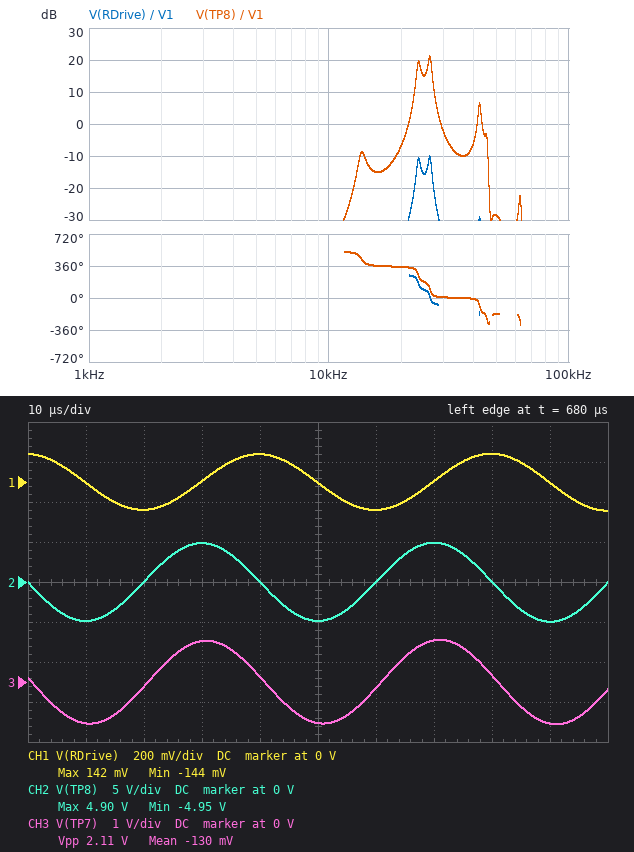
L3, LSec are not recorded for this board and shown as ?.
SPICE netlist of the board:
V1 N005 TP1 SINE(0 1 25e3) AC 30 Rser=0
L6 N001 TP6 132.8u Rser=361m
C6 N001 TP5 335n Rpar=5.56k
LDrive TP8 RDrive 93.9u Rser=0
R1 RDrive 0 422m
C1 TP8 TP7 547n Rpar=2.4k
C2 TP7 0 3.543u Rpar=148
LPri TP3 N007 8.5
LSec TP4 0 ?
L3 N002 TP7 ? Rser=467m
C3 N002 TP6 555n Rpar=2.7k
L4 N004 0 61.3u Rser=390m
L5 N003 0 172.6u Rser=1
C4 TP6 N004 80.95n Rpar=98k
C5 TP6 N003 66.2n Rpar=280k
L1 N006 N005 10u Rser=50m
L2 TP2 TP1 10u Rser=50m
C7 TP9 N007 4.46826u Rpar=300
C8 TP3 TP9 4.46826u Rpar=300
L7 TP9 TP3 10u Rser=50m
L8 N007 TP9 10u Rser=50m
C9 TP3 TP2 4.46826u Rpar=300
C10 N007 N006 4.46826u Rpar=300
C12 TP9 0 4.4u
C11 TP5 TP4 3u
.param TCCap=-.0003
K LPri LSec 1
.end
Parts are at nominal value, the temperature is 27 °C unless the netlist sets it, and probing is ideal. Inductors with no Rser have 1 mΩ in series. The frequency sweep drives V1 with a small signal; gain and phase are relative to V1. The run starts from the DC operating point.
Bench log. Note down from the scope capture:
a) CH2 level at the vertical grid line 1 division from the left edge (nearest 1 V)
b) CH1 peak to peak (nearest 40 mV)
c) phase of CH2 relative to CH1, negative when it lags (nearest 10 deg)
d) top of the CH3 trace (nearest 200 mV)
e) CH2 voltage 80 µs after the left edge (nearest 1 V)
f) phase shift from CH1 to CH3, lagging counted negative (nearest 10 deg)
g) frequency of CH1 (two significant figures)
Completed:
-5 V
280 mV
90 deg
1.0 V
0 V
80 deg
25 kHz
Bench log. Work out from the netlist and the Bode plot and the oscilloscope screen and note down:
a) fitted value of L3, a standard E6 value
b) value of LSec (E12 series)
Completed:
47 µH
39 H
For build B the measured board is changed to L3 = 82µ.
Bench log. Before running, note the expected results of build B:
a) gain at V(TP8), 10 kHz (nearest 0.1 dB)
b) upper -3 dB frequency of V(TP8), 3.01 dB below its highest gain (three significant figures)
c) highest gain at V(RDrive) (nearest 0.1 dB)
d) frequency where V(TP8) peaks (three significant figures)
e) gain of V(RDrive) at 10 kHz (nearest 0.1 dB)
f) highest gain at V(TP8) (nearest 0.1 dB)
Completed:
-39.9 dB
25.6 kHz
-6.7 dB
25.2 kHz
-62.9 dB
24.3 dB
